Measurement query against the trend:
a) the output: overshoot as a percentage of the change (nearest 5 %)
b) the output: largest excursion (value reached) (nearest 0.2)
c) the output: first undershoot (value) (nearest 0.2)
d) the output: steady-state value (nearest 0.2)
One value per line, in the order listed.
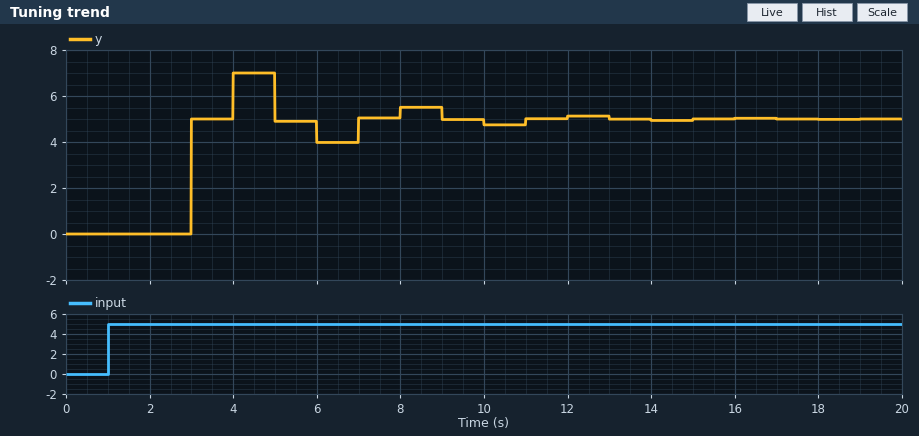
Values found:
40 %
7.0
4.0
5.0
